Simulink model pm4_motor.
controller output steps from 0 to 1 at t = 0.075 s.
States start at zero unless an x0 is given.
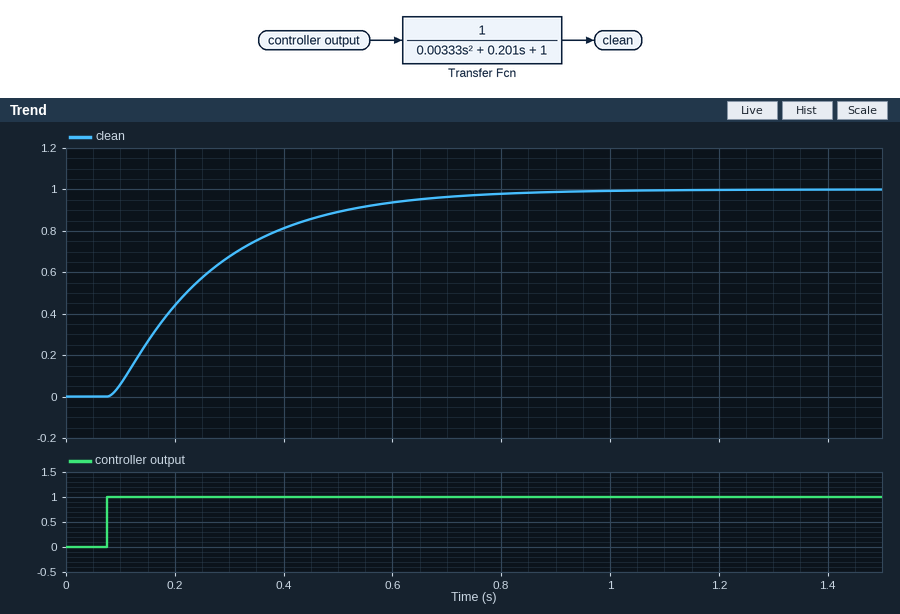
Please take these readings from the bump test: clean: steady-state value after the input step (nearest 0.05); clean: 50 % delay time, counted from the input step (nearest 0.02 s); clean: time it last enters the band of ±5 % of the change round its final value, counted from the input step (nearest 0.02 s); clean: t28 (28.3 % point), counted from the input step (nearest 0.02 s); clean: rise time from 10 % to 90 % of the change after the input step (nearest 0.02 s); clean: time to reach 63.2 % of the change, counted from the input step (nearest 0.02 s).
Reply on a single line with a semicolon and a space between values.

1.00; 0.14 s; 0.56 s; 0.08 s; 0.40 s; 0.20 s
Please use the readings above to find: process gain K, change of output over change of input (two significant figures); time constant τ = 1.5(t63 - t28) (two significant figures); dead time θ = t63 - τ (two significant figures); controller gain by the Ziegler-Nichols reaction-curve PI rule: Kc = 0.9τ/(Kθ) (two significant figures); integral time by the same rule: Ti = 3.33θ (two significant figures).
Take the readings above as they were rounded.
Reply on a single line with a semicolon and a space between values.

1.0; 0.18 s; 0.020 s; 8.1; 0.067 s
